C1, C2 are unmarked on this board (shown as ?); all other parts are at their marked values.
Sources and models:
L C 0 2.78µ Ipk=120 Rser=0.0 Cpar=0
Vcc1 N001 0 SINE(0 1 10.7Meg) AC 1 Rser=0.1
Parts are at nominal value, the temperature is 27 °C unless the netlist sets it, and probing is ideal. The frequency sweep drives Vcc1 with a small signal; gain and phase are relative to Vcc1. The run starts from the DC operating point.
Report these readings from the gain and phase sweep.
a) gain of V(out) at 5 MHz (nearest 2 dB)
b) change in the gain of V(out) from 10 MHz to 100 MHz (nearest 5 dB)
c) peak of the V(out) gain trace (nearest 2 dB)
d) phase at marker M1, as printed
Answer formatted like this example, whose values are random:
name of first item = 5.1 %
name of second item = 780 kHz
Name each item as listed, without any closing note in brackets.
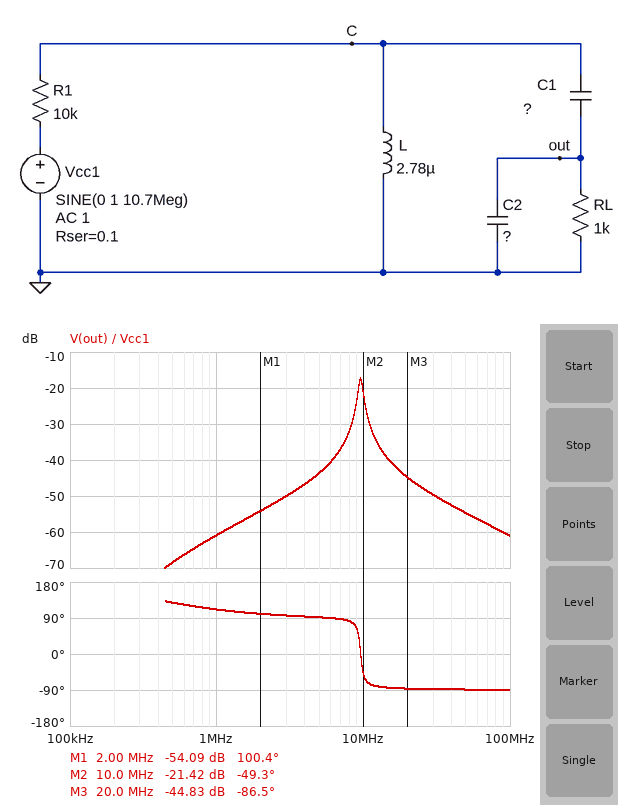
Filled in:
gain of V(out) at 5 MHz = -44 dB
change in the gain of V(out) from 10 MHz to 100 MHz = -40 dB
peak of the V(out) gain trace = -18 dB
phase at marker M1, as printed = 100.4 deg
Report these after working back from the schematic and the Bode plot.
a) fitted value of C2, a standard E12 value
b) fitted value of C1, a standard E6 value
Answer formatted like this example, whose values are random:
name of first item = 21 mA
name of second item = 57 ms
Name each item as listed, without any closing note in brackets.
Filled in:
fitted value of C2, a standard E12 value = 180 pF
fitted value of C1, a standard E6 value = 220 pF
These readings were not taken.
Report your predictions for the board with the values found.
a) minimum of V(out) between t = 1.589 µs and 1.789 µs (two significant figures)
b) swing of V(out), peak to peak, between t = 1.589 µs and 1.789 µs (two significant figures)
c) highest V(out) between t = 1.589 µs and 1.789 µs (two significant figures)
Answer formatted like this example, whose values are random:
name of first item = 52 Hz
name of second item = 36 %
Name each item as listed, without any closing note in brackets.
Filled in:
minimum of V(out) between t = 1.589 µs and 1.789 µs = -39 mV
swing of V(out), peak to peak, between t = 1.589 µs and 1.789 µs = 78 mV
highest V(out) between t = 1.589 µs and 1.789 µs = 39 mV
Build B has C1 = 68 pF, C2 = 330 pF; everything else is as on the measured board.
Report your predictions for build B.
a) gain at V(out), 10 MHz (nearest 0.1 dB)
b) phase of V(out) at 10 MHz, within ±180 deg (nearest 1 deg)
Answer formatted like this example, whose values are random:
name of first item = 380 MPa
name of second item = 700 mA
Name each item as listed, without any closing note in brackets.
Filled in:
gain at V(out), 10 MHz = -42.1 dB
phase of V(out) at 10 MHz, within ±180 deg = 89 deg
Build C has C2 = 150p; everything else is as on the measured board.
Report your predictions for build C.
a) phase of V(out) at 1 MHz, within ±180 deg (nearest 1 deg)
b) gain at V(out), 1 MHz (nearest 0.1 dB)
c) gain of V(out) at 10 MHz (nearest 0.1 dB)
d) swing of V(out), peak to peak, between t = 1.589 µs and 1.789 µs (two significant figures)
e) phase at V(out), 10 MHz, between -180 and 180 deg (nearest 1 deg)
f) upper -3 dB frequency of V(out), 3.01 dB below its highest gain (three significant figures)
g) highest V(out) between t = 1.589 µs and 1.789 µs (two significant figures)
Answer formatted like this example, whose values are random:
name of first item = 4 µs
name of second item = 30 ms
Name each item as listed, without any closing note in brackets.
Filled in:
phase of V(out) at 1 MHz, within ±180 deg = 113 deg
gain at V(out), 1 MHz = -60.3 dB
gain of V(out) at 10 MHz = -17.9 dB
swing of V(out), peak to peak, between t = 1.589 µs and 1.789 µs = 150 mV
phase at V(out), 10 MHz, between -180 and 180 deg = 16 deg
upper -3 dB frequency of V(out), 3.01 dB below its highest gain = 10.5 MHz
highest V(out) between t = 1.589 µs and 1.789 µs = 73 mV
